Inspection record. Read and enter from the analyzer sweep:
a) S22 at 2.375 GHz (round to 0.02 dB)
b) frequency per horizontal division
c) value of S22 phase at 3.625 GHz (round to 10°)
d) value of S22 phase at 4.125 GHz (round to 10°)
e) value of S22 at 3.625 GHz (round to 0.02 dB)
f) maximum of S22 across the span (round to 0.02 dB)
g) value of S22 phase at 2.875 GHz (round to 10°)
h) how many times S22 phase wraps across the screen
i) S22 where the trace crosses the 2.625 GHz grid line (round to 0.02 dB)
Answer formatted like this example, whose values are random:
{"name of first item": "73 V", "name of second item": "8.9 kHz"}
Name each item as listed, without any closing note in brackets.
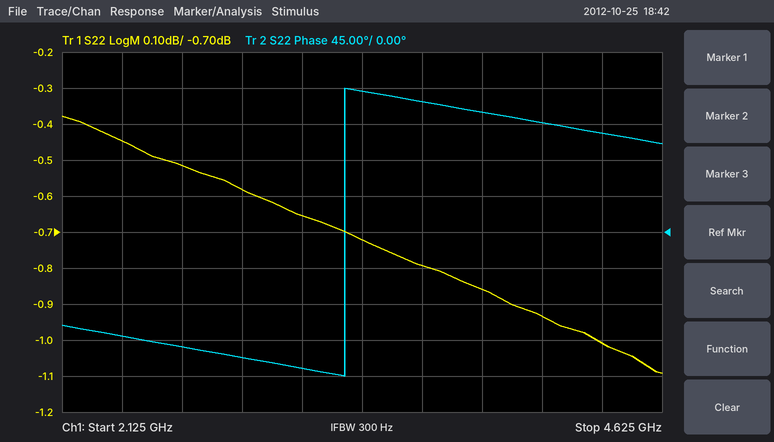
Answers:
{"S22 at 2.375 GHz": "-0.44 dB", "frequency per horizontal division": "250 MHz", "value of S22 phase at 3.625 GHz": "160°", "value of S22 phase at 4.125 GHz": "140°", "value of S22 at 3.625 GHz": "-0.80 dB", "maximum of S22 across the span": "-0.38 dB", "value of S22 phase at 2.875 GHz": "-160°", "how many times S22 phase wraps across the screen": "1", "S22 where the trace crosses the 2.625 GHz grid line": "-0.52 dB"}
